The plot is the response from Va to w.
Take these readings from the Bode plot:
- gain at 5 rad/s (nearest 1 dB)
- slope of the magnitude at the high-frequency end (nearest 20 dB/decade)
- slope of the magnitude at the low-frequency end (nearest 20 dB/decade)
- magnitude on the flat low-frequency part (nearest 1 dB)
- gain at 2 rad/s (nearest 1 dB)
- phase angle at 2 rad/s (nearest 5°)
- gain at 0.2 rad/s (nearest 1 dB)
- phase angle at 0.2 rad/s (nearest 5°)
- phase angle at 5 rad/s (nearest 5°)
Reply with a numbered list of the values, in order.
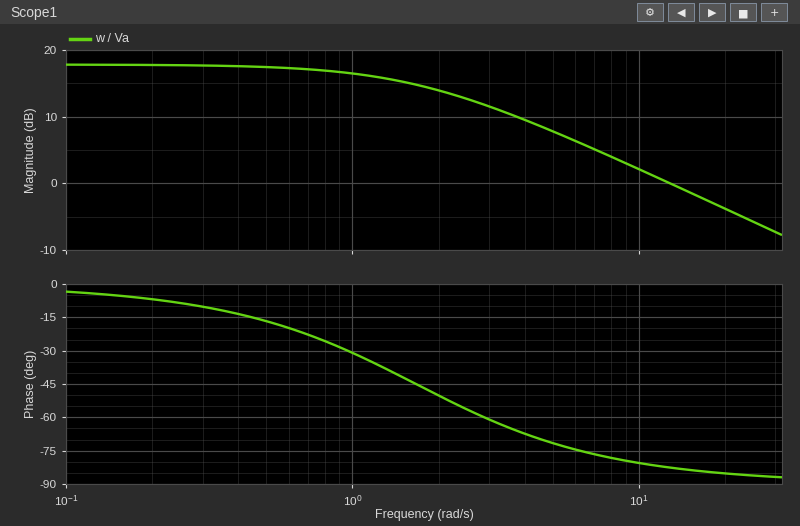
1. 8 dB
2. -20 dB/decade
3. 0 dB/decade
4. 18 dB
5. 14 dB
6. -50°
7. 18 dB
8. -5°
9. -70°
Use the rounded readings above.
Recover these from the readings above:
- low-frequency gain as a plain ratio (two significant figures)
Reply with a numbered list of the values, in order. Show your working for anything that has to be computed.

1. 10^(18 / 20) = 7.9
